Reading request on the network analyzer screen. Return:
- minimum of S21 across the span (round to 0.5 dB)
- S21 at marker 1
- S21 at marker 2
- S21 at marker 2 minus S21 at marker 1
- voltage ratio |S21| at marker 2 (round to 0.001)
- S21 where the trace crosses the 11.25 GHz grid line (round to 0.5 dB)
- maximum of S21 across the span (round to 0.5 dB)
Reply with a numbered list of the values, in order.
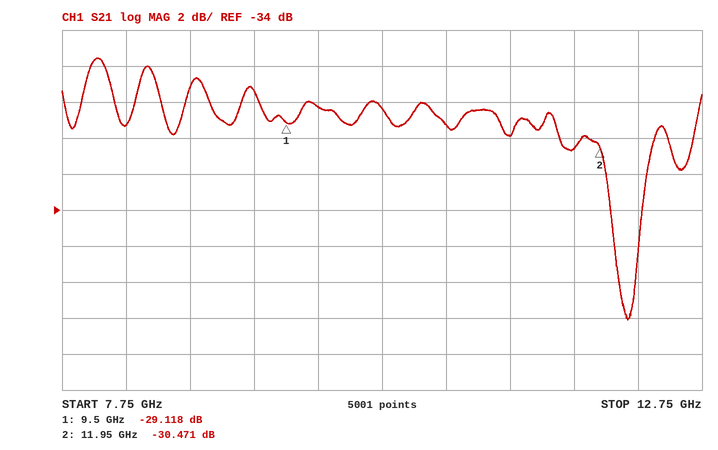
1. -40.0 dB
2. -29.118 dB
3. -30.471 dB
4. -1.353 dB
5. 0.030
6. -30.0 dB
7. -25.5 dB
